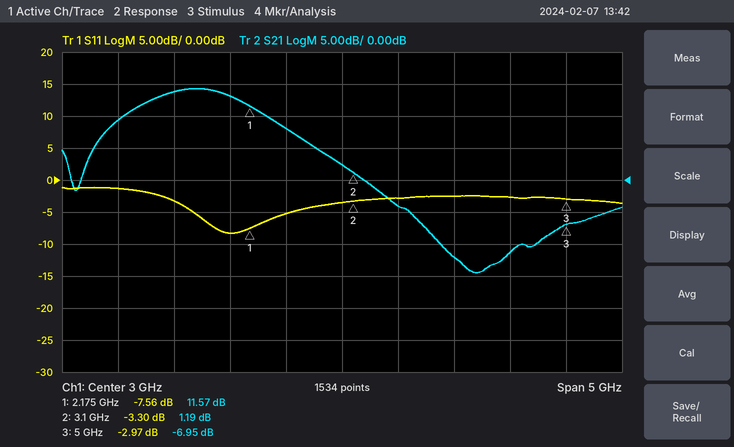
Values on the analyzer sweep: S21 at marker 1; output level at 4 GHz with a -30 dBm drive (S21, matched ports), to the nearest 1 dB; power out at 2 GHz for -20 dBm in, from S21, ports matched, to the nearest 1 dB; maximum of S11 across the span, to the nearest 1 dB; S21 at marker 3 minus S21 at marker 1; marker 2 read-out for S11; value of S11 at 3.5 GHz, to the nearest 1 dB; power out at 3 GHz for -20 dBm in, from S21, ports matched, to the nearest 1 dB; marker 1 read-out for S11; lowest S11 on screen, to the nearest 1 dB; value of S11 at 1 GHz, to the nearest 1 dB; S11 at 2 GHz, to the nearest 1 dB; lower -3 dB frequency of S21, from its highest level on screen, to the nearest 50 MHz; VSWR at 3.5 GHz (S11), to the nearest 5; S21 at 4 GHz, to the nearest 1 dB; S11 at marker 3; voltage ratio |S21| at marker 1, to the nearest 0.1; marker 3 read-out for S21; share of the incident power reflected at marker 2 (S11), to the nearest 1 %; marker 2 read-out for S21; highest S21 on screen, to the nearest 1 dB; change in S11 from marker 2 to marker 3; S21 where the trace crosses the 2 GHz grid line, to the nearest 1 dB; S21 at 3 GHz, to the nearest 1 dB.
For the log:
11.57 dB
-42 dBm
-7 dBm
-1 dB
-18.52 dB
-3.30 dB
-3 dB
-18 dBm
-7.56 dB
-8 dB
-1 dB
-8 dB
1.15 GHz
5
-12 dB
-2.97 dB
3.8
-6.95 dB
47 %
1.19 dB
14 dB
0.33 dB
13 dB
2 dB
